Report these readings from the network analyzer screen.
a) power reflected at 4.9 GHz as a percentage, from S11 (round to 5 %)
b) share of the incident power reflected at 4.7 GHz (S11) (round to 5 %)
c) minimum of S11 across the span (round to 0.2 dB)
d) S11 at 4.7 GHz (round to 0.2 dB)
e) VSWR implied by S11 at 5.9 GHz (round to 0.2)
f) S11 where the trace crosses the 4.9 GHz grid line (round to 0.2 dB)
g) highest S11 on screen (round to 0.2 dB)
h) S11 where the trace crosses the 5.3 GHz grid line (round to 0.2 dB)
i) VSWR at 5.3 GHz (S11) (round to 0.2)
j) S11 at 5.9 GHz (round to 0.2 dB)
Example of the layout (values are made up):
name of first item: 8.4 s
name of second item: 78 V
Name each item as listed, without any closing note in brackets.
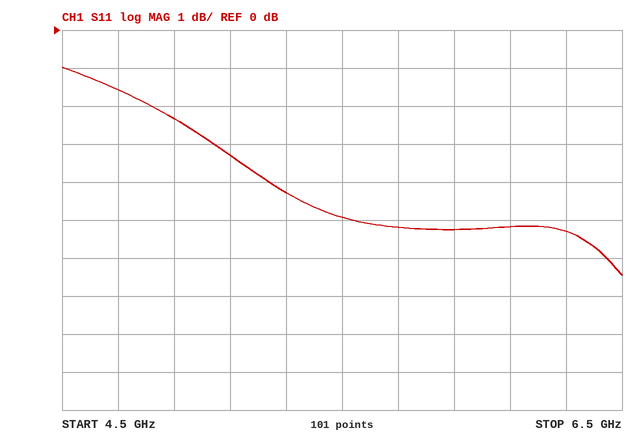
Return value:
power reflected at 4.9 GHz as a percentage, from S11: 60 %
share of the incident power reflected at 4.7 GHz (S11): 70 %
minimum of S11 across the span: -6.4 dB
S11 at 4.7 GHz: -1.6 dB
VSWR implied by S11 at 5.9 GHz: 3.4
S11 where the trace crosses the 4.9 GHz grid line: -2.4 dB
highest S11 on screen: -1.0 dB
S11 where the trace crosses the 5.3 GHz grid line: -4.2 dB
VSWR at 5.3 GHz (S11): 4.2
S11 at 5.9 GHz: -5.2 dB
